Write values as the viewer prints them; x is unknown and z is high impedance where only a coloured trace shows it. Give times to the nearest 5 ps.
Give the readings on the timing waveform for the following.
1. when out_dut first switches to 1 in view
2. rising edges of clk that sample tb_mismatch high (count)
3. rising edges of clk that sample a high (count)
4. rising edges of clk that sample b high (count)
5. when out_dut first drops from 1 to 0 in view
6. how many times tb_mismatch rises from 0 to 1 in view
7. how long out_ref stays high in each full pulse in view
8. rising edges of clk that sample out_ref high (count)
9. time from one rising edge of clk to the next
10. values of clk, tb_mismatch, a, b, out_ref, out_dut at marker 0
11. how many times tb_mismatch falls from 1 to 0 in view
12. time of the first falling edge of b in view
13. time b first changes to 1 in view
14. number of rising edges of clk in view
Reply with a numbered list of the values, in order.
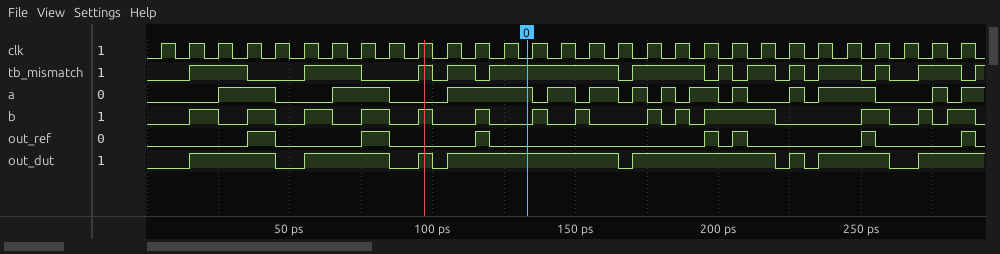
1. 15 ps
2. 18
3. 14
4. 10
5. 45 ps
6. 13
7. 10 ps, 10 ps, 5 ps, 5 ps, 5 ps, 5 ps, 5 ps
8. 3
9. 10 ps
10. clk=0, tb_mismatch=1, a=1, b=0, out_ref=0, out_dut=1
11. 12
12. 25 ps
13. 15 ps
14. 29
